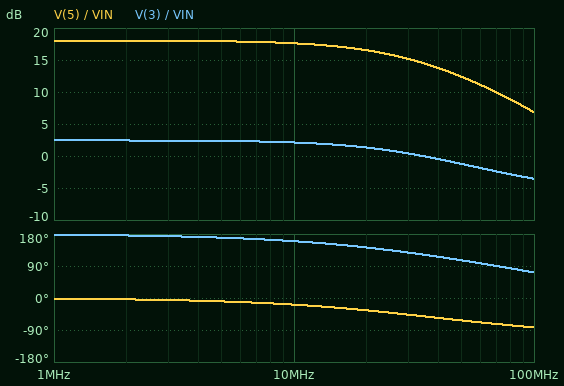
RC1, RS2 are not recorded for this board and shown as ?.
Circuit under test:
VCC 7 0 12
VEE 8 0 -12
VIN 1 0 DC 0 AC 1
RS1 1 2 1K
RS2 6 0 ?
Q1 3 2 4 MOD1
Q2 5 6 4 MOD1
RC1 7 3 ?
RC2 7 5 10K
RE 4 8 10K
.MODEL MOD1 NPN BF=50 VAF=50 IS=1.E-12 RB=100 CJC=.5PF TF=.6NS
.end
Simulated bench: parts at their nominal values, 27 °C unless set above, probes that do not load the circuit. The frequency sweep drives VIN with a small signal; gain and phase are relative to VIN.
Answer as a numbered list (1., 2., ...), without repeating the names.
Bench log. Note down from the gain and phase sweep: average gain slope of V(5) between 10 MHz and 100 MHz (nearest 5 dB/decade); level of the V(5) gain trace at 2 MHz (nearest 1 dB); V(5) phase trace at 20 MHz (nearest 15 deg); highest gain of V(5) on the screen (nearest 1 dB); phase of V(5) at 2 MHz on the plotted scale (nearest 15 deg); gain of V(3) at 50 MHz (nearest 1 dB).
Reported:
1. -10 dB/decade
2. 18 dB
3. -30 deg
4. 18 dB
5. 0 deg
6. -1 dB
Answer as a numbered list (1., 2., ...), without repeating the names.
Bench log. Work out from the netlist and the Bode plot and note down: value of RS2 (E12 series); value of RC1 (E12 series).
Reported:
1. 680 Ω
2. 33 kΩ
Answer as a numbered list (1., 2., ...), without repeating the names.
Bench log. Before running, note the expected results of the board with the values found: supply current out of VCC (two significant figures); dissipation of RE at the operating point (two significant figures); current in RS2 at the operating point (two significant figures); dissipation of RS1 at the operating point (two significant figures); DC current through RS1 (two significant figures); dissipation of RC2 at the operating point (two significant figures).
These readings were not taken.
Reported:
1. 1.1 mA
2. 13 mW
3. 13 µA
4. 450 nW
5. 21 µA
6. 5.4 mW
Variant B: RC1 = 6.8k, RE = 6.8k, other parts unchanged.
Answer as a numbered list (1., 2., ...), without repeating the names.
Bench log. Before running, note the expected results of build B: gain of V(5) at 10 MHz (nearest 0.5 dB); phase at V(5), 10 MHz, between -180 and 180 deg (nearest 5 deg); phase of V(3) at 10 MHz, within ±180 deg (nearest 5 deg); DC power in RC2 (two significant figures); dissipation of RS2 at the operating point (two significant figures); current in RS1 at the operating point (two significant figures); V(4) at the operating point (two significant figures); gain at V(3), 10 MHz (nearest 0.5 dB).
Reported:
1. 29.0 dB
2. -75 deg
3. 110 deg
4. 7.3 mW
5. 170 nW
6. 14 µA
7. -540 mV
8. 26.0 dB
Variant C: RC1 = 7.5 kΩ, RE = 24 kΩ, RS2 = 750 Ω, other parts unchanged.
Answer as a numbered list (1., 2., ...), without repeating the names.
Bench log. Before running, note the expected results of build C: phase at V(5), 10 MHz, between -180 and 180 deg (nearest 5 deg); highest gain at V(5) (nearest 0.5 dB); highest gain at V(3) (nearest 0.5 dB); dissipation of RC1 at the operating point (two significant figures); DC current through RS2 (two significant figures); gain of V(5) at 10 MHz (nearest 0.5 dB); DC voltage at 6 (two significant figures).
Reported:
1. -55 deg
2. 31.5 dB
3. 29.0 dB
4. 410 µW
5. 4.0 µA
6. 27.5 dB
7. -3.0 mV
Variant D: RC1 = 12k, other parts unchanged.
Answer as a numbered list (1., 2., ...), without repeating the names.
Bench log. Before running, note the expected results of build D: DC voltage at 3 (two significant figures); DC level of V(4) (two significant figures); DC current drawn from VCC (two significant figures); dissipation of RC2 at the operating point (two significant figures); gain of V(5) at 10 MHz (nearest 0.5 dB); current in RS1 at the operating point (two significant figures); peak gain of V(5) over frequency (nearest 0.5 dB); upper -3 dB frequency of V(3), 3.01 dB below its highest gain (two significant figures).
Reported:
1. 5.6 V
2. -530 mV
3. 1.1 mA
4. 3.5 mW
5. 27.0 dB
6. 9.6 µA
7. 37.0 dB
8. 3.4 MHz
